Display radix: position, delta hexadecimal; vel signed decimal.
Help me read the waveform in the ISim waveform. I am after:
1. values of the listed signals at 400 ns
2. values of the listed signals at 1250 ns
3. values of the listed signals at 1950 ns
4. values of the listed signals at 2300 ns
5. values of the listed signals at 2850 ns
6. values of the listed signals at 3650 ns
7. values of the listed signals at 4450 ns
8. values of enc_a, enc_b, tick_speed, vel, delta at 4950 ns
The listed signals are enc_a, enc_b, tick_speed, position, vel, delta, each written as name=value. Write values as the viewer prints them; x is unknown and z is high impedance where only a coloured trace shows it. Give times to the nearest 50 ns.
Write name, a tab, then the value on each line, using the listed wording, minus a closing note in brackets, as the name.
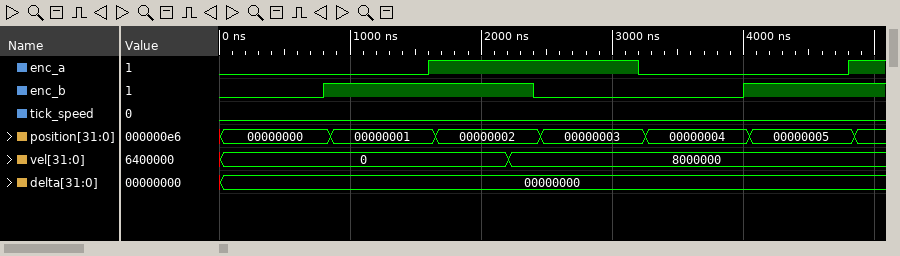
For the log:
values of the listed signals at 400 ns	enc_a=0, enc_b=0, tick_speed=0, position=00000000, vel=0, delta=00000000
values of the listed signals at 1250 ns	enc_a=0, enc_b=1, tick_speed=0, position=00000001, vel=0, delta=00000000
values of the listed signals at 1950 ns	enc_a=1, enc_b=1, tick_speed=0, position=00000002, vel=0, delta=00000000
values of the listed signals at 2300 ns	enc_a=1, enc_b=1, tick_speed=0, position=00000002, vel=8000000, delta=00000000
values of the listed signals at 2850 ns	enc_a=1, enc_b=0, tick_speed=0, position=00000003, vel=8000000, delta=00000000
values of the listed signals at 3650 ns	enc_a=0, enc_b=0, tick_speed=0, position=00000004, vel=8000000, delta=00000000
values of the listed signals at 4450 ns	enc_a=0, enc_b=1, tick_speed=0, position=00000005, vel=8000000, delta=00000000
values of enc_a, enc_b, tick_speed, vel, delta at 4950 ns	enc_a=1, enc_b=1, tick_speed=0, vel=8000000, delta=00000000
